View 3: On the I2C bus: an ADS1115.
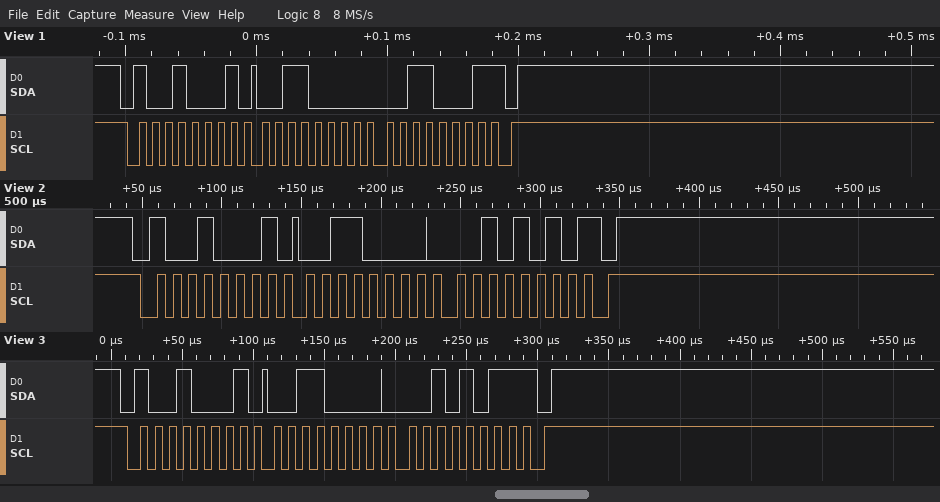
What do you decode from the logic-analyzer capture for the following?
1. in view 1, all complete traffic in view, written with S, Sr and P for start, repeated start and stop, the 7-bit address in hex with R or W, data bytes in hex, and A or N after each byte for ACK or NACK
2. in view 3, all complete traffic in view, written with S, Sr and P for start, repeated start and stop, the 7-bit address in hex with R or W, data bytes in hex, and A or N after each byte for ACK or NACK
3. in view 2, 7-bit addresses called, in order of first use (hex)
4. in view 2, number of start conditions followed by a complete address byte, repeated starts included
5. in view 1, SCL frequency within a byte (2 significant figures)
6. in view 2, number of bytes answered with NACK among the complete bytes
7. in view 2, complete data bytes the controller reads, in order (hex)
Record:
S 48R A 30 A 31 N P
S 48R A 30 A 2B N P
0x48
1
100 kHz
1
30 2A
